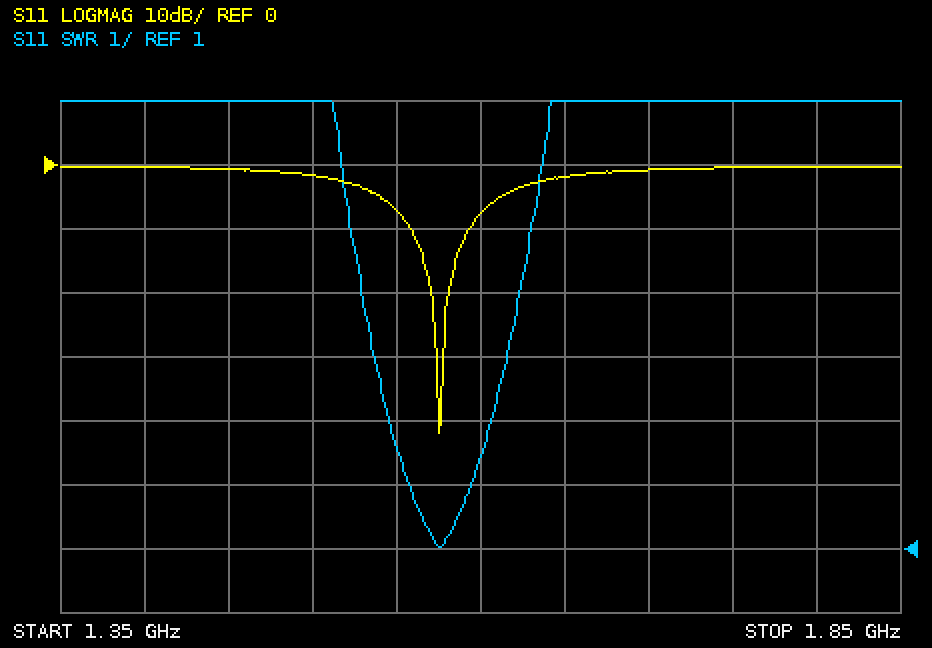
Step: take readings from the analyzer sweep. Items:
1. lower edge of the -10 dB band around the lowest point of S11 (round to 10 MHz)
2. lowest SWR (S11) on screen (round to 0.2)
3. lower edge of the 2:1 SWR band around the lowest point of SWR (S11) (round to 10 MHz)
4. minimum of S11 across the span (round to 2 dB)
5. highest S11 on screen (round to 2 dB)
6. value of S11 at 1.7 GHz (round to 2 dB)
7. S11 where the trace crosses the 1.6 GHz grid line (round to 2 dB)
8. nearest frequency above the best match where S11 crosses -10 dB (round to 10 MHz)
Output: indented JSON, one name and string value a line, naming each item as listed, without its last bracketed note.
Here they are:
{
  "lower edge of the -10 dB band around the lowest point of S11": "1.56 GHz",
  "lowest SWR (S11) on screen": "1.0",
  "lower edge of the 2:1 SWR band around the lowest point of SWR (S11)": "1.56 GHz",
  "minimum of S11 across the span": "-42 dB",
  "highest S11 on screen": "0 dB",
  "value of S11 at 1.7 GHz": "0 dB",
  "S11 where the trace crosses the 1.6 GHz grid line": "-8 dB",
  "nearest frequency above the best match where S11 crosses -10 dB": "1.59 GHz"
}
